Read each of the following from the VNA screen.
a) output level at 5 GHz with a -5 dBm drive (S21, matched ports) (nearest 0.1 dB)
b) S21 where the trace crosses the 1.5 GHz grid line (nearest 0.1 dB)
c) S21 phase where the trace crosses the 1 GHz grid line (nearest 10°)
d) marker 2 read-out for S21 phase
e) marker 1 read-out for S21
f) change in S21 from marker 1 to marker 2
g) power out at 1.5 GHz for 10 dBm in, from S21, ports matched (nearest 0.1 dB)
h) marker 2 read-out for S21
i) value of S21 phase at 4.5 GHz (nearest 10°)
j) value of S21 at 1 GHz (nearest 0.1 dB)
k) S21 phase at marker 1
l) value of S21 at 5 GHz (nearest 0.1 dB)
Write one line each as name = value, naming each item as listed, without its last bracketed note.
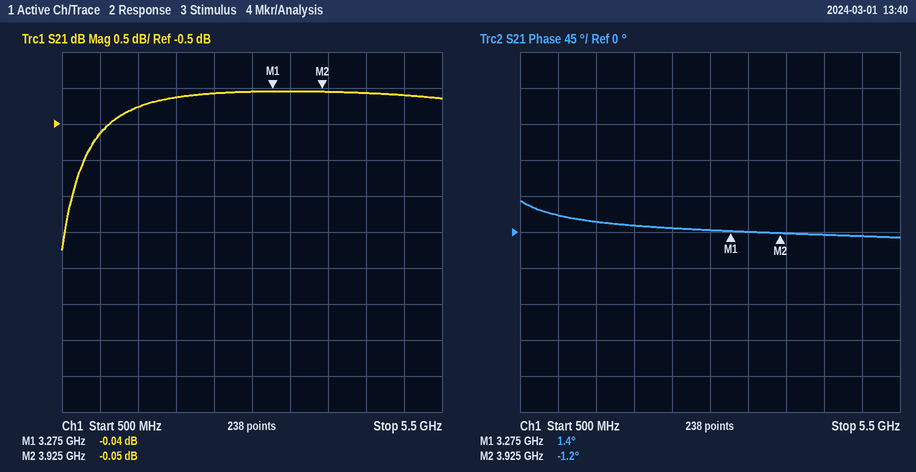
output level at 5 GHz with a -5 dBm drive (S21, matched ports) = -5.1 dBm
S21 where the trace crosses the 1.5 GHz grid line = -0.3 dB
S21 phase where the trace crosses the 1 GHz grid line = 20°
marker 2 read-out for S21 phase = -1.2°
marker 1 read-out for S21 = -0.04 dB
change in S21 from marker 1 to marker 2 = -0.01 dB
power out at 1.5 GHz for 10 dBm in, from S21, ports matched = 9.7 dBm
marker 2 read-out for S21 = -0.05 dB
value of S21 phase at 4.5 GHz = 0°
value of S21 at 1 GHz = -0.6 dB
S21 phase at marker 1 = 1.4°
value of S21 at 5 GHz = -0.1 dB
